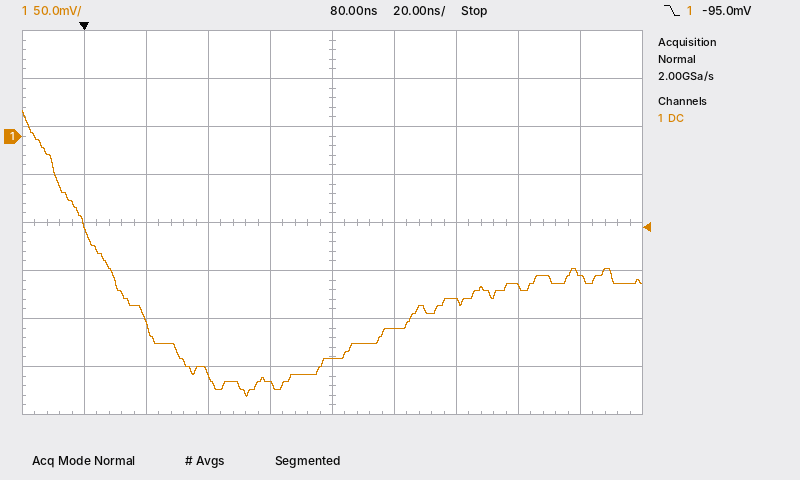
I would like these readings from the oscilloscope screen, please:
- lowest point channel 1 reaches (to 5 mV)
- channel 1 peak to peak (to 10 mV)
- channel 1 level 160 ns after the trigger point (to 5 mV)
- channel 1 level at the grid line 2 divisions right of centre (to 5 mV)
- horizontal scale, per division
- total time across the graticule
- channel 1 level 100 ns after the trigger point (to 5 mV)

-270 mV
300 mV
-145 mV
-170 mV
20 ns
200 ns
-200 mV
